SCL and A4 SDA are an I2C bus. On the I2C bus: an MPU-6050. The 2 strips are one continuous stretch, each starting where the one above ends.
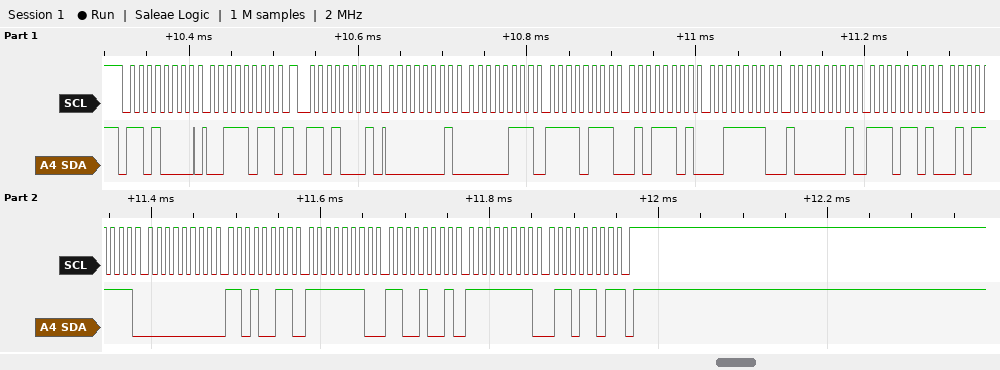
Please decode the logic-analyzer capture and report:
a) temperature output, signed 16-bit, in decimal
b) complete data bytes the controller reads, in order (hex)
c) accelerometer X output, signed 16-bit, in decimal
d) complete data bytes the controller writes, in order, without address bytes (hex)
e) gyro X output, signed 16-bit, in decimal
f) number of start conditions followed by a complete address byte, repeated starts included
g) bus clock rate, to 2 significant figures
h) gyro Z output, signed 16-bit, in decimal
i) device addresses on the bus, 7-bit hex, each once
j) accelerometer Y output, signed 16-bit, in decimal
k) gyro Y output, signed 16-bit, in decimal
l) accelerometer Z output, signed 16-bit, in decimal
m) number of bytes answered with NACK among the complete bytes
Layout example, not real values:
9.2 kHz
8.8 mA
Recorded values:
-4769
01 07 F7 5D 3E 81 ED 5F 00 D3 FE C9 FF 6D
263
3B
211
2
100 kHz
-147
0x68
-2211
-311
16001
1
